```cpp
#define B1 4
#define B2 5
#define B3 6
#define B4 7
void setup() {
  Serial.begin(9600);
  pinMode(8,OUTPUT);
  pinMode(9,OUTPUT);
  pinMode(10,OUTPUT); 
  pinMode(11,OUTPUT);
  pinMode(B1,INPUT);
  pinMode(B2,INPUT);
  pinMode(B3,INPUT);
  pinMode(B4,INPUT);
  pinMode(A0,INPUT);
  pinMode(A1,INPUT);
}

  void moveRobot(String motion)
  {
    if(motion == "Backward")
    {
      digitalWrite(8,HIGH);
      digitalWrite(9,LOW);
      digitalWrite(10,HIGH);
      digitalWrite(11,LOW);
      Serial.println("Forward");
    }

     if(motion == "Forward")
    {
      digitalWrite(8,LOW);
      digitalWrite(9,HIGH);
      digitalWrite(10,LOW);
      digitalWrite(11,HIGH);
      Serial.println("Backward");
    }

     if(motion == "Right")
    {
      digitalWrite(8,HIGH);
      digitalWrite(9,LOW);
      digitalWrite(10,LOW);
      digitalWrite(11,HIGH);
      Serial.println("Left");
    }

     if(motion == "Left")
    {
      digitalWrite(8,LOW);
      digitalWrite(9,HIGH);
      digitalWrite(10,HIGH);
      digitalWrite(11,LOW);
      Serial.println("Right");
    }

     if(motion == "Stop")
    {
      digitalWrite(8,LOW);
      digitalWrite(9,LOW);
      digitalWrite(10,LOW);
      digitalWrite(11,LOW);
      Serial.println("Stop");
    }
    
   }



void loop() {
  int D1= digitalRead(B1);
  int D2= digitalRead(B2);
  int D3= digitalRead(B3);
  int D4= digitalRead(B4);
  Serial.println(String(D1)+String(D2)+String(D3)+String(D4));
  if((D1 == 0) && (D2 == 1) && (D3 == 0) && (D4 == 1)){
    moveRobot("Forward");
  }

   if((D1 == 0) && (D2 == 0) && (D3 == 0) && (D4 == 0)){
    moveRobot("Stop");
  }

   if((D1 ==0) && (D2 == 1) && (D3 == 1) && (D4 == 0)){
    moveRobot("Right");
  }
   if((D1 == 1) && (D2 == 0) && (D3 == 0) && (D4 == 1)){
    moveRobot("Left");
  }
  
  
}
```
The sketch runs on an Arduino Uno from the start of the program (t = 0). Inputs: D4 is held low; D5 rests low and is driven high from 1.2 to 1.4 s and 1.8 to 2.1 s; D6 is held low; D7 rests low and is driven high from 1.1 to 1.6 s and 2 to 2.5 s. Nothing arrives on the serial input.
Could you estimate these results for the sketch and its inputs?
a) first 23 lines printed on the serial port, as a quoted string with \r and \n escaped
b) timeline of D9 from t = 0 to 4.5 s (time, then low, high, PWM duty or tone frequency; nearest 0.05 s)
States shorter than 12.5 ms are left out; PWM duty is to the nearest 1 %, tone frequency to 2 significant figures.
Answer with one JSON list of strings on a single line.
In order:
["\"0000\\r\\nStop\\r\\n0000\\r\\nStop\\r\\n0000\\r\\nStop\\r\\n0000\\r\\nStop\\r\\n0000\\r\\nStop\\r\\n0000\\r\\nStop\\r\\n0000\\r\\nStop\\r\\n0000\\r\\nStop\\r\\n0000\\r\\nStop\\r\\n0000\\r\\nStop\\r\\n0000\\r\\nStop\\r\\n0000\\r\\n\"", "0 s low; 1.2 s high; 1.6 s low; 2 s high; 2.5 s low"]
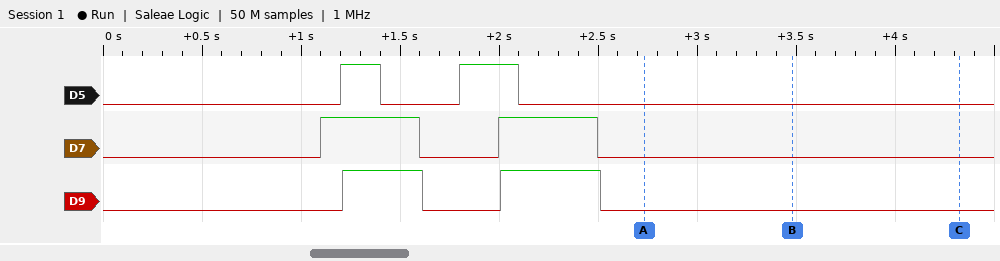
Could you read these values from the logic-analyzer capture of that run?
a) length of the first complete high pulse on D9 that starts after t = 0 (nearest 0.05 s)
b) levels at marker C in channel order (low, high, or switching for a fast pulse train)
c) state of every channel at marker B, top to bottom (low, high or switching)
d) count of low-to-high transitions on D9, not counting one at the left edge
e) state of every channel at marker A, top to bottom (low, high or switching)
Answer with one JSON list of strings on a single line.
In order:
["0.40 s", "D5 low, D7 low, D9 low", "D5 low, D7 low, D9 low", "2", "D5 low, D7 low, D9 low"]
